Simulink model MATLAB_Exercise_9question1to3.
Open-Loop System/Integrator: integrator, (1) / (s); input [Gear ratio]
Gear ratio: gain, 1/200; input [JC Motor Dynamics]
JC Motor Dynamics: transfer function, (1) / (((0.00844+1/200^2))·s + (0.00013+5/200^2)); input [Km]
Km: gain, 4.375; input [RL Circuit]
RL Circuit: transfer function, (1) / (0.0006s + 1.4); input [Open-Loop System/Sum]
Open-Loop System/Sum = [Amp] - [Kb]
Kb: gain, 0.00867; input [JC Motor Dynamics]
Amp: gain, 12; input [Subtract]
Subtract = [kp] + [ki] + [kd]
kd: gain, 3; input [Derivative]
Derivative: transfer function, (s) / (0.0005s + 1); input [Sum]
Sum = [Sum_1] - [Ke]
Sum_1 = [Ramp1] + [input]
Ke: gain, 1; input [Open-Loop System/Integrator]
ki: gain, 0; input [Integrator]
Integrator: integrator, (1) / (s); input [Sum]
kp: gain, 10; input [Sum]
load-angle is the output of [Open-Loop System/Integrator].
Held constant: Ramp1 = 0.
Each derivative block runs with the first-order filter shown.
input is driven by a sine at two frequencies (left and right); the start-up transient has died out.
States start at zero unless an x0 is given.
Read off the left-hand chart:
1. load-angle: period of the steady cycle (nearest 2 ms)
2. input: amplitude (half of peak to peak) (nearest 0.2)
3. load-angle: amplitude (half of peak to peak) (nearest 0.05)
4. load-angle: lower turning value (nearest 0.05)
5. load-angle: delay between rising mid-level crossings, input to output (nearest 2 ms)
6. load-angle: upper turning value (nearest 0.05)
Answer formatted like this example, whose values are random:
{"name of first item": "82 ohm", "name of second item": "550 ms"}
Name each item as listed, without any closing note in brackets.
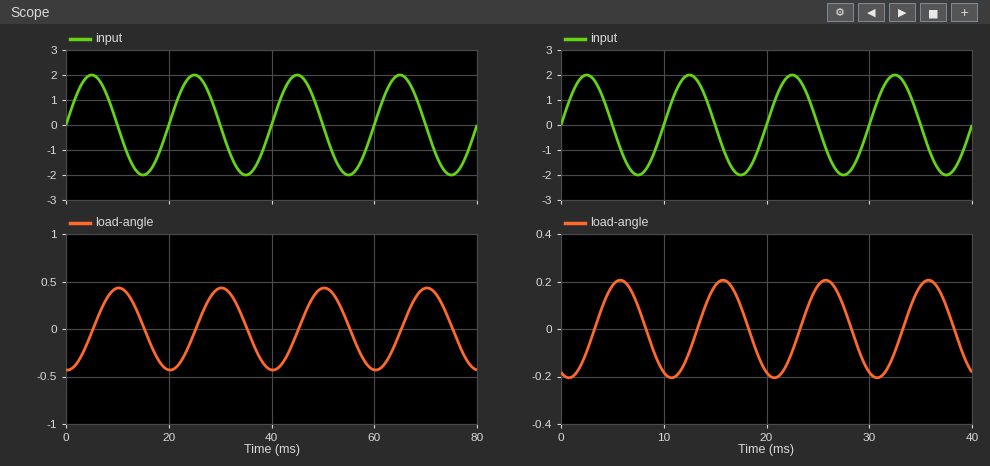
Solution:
{"load-angle: period of the steady cycle": "20 ms", "input: amplitude (half of peak to peak)": "2.0", "load-angle: amplitude (half of peak to peak)": "0.45", "load-angle: lower turning value": "-0.45", "load-angle: delay between rising mid-level crossings, input to output": "6 ms", "load-angle: upper turning value": "0.45"}
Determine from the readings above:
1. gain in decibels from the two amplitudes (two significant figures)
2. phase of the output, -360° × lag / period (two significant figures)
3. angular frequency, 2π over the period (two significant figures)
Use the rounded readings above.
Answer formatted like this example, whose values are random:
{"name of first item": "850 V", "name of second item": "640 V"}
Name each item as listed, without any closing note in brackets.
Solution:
{"gain in decibels from the two amplitudes": "-13 dB", "phase of the output, -360° × lag / period": "-110°", "angular frequency, 2π over the period": "0.31 rad/ms"}
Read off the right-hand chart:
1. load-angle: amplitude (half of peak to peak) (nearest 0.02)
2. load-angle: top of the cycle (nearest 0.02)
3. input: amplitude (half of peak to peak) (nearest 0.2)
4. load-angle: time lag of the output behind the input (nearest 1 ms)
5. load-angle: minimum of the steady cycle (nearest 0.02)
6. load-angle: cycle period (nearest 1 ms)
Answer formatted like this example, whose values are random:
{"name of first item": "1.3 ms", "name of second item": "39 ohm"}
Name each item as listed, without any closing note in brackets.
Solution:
{"load-angle: amplitude (half of peak to peak)": "0.20", "load-angle: top of the cycle": "0.20", "input: amplitude (half of peak to peak)": "2.0", "load-angle: time lag of the output behind the input": "3 ms", "load-angle: minimum of the steady cycle": "-0.20", "load-angle: cycle period": "10 ms"}
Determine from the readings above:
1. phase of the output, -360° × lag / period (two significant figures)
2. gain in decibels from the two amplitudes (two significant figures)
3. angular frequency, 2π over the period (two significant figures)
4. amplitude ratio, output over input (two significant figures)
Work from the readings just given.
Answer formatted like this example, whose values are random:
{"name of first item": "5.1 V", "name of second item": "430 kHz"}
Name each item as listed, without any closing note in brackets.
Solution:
{"phase of the output, -360° × lag / period": "-110°", "gain in decibels from the two amplitudes": "-20 dB", "angular frequency, 2π over the period": "0.63 rad/ms", "amplitude ratio, output over input": "0.10"}
